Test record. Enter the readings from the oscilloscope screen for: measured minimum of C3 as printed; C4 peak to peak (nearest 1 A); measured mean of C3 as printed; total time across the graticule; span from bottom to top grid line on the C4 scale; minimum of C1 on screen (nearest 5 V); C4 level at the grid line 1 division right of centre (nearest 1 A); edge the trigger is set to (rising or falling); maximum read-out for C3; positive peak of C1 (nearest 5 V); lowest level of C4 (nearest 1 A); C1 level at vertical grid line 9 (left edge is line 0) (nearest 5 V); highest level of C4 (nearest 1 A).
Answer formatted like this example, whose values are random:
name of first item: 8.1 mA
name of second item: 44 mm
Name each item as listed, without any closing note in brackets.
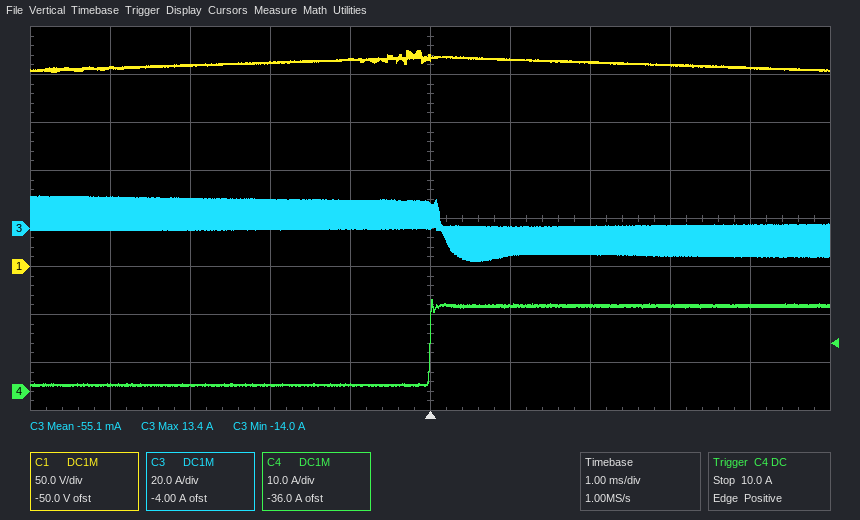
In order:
measured minimum of C3 as printed: -14.0 A
C4 peak to peak: 18 A
measured mean of C3 as printed: -55.1 mA
total time across the graticule: 10 ms
span from bottom to top grid line on the C4 scale: 80 A
minimum of C1 on screen: 200 V
C4 level at the grid line 1 division right of centre: 18 A
edge the trigger is set to: rising
maximum read-out for C3: 13.4 A
positive peak of C1: 225 V
lowest level of C4: 1 A
C1 level at vertical grid line 9 (left edge is line 0): 205 V
highest level of C4: 19 A
